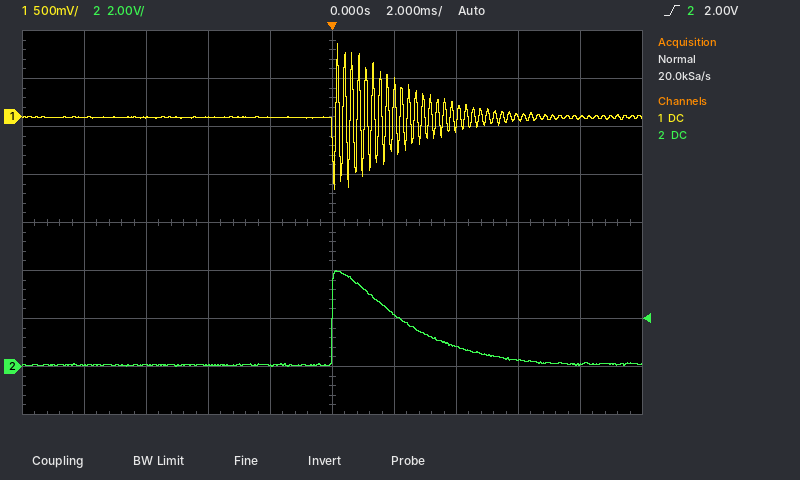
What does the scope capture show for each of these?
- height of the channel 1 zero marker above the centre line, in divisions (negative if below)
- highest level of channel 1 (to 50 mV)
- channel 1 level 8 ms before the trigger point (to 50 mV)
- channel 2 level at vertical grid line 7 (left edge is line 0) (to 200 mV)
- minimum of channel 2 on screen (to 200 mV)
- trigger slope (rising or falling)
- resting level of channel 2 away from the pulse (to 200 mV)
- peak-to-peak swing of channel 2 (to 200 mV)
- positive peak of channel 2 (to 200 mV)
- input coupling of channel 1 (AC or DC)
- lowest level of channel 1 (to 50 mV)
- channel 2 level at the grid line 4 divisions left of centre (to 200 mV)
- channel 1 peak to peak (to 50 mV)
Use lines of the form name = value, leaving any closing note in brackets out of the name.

height of the channel 1 zero marker above the centre line, in divisions = +2.2 div
highest level of channel 1 = 750 mV
channel 1 level 8 ms before the trigger point = 0 mV
channel 2 level at vertical grid line 7 (left edge is line 0) = 800 mV
minimum of channel 2 on screen = 0.0 V
trigger slope = rising
resting level of channel 2 away from the pulse = 0.0 V
peak-to-peak swing of channel 2 = 4.0 V
positive peak of channel 2 = 4.0 V
input coupling of channel 1 = DC
lowest level of channel 1 = -750 mV
channel 2 level at the grid line 4 divisions left of centre = 0.0 V
channel 1 peak to peak = 1.50 V
